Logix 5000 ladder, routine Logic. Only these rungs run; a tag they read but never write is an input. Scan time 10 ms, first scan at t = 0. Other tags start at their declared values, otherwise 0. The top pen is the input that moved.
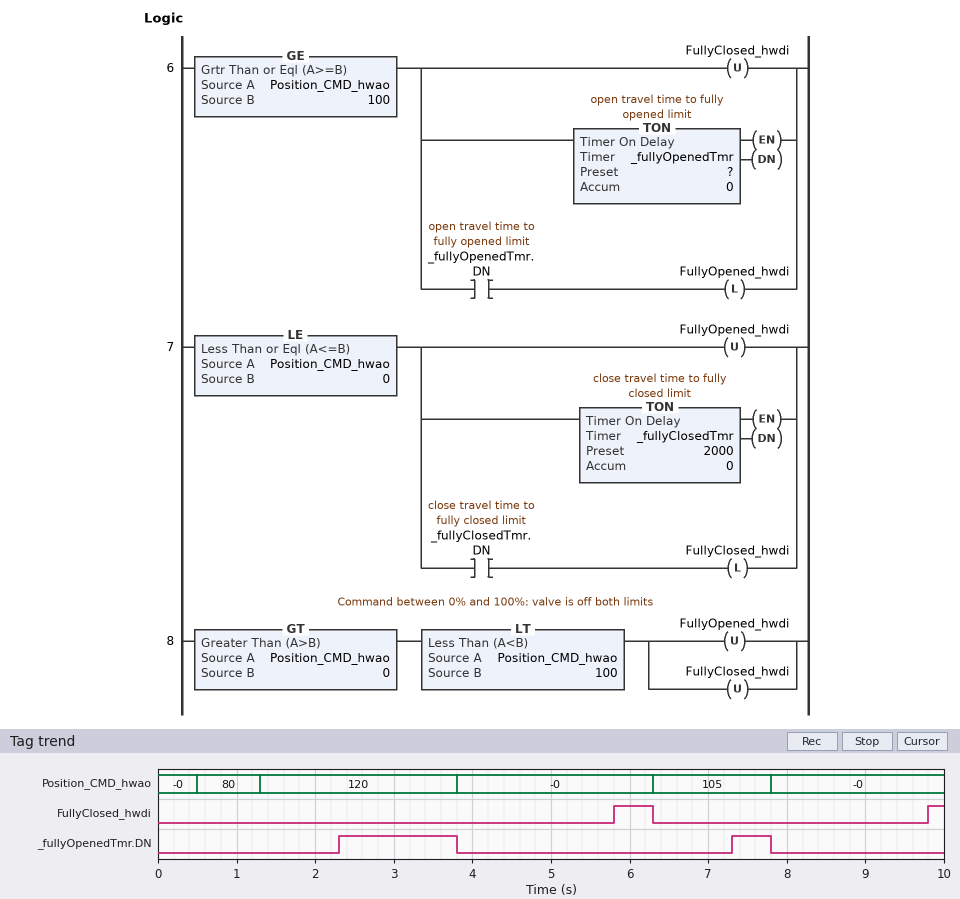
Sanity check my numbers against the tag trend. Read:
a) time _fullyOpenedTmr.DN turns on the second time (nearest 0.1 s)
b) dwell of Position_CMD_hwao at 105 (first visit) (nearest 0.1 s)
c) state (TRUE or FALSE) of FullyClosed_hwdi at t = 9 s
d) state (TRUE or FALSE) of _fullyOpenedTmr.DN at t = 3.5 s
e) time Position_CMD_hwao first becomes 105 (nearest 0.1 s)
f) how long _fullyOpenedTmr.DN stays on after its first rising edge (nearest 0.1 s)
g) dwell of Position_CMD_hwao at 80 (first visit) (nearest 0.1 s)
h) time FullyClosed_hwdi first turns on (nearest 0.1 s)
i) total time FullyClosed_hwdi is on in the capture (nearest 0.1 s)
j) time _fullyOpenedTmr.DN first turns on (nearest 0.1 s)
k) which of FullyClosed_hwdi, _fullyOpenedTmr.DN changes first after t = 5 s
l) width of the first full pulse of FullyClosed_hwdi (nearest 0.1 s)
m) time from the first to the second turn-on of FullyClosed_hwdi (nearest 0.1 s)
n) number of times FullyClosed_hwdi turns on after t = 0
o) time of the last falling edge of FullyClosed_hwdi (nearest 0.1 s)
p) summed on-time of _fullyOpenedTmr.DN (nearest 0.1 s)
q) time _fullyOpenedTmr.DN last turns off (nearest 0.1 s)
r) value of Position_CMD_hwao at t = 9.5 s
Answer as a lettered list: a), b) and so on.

a) 7.3 s
b) 1.5 s
c) FALSE
d) TRUE
e) 6.3 s
f) 1.5 s
g) 0.8 s
h) 5.8 s
i) 0.7 s
j) 2.3 s
k) FullyClosed_hwdi
l) 0.5 s
m) 4.0 s
n) 2
o) 6.3 s
p) 2.0 s
q) 7.8 s
r) -0
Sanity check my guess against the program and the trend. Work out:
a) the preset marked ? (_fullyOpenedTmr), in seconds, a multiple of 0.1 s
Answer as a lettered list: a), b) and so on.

a) 1.0 s
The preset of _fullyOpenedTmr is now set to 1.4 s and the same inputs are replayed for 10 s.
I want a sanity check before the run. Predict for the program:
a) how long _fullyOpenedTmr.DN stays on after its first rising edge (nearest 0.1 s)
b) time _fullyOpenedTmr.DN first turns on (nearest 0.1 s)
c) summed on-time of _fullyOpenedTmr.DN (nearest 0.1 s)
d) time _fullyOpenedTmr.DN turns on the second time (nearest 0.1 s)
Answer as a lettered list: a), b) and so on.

a) 1.1 s
b) 2.7 s
c) 1.2 s
d) 7.7 s
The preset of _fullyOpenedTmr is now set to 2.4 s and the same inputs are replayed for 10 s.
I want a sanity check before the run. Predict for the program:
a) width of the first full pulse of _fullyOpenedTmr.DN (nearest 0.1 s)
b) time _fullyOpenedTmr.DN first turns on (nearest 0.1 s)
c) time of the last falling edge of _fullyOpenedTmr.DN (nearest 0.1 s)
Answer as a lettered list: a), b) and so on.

a) 0.1 s
b) 3.7 s
c) 3.8 s
